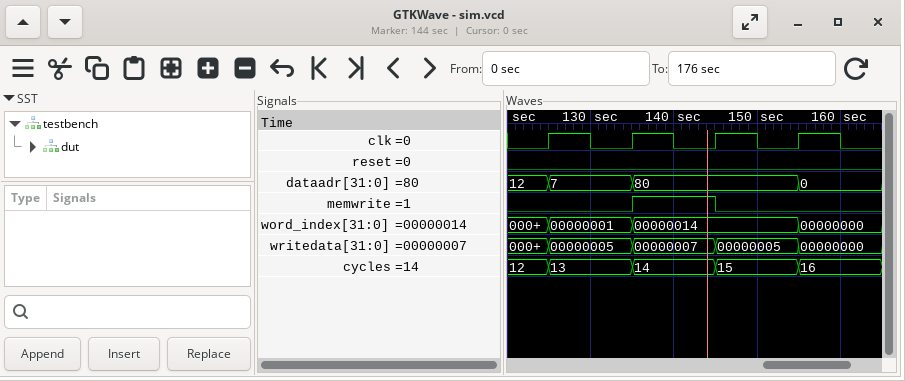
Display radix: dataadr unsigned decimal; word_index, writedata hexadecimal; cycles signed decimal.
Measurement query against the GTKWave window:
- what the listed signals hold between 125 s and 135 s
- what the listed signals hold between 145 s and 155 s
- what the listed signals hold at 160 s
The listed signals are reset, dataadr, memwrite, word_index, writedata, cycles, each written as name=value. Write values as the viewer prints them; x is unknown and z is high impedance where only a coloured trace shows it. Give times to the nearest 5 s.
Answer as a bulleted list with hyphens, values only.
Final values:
- reset=0, dataadr=7, memwrite=0, word_index=00000001, writedata=00000005, cycles=13
- reset=0, dataadr=80, memwrite=0, word_index=00000014, writedata=00000005, cycles=15
- reset=0, dataadr=0, memwrite=0, word_index=00000000, writedata=00000000, cycles=16
